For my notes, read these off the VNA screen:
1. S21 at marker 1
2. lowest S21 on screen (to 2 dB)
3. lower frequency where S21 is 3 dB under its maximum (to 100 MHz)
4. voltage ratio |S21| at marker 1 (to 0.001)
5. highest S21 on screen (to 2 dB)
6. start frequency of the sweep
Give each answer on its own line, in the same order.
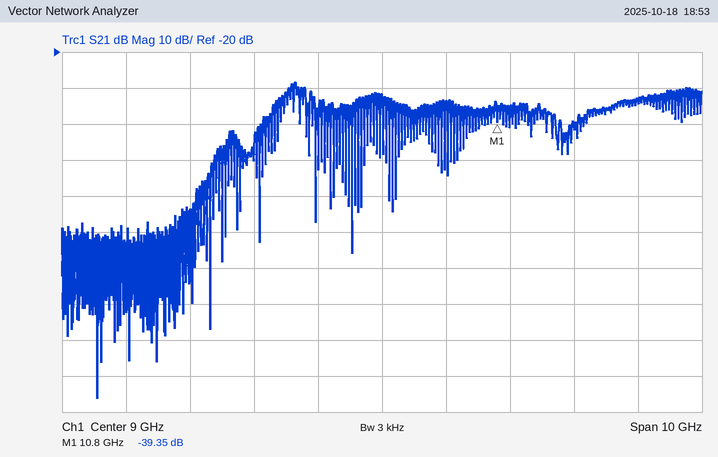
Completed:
-39.35 dB
-116 dB
7.6 GHz
0.011
-28 dB
4 GHz
